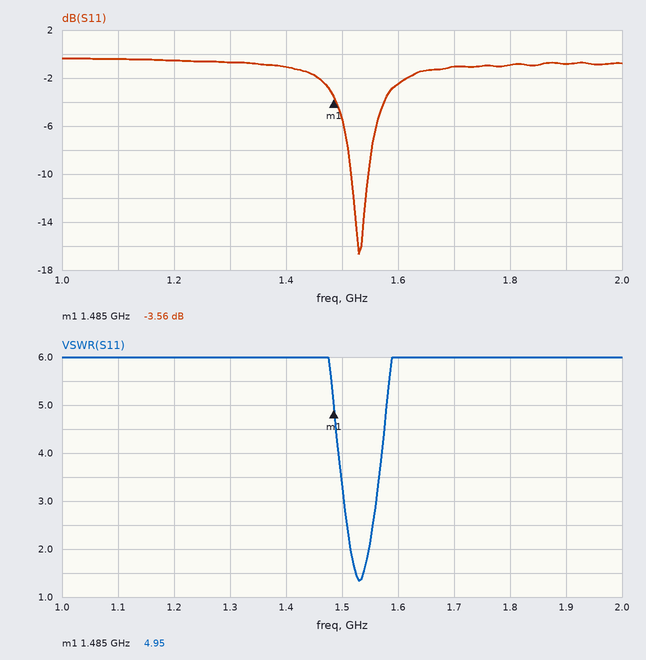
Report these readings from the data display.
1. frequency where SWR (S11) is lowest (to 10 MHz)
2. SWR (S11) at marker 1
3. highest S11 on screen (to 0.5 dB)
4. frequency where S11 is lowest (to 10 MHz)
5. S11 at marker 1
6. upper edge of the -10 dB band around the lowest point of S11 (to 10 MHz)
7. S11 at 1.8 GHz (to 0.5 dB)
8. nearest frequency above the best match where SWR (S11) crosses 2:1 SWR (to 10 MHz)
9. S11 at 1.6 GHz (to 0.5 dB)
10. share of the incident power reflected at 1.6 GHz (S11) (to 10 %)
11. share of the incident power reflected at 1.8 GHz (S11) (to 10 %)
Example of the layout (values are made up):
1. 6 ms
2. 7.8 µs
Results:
1. 1.53 GHz
2. 4.95
3. -0.5 dB
4. 1.53 GHz
5. -3.56 dB
6. 1.55 GHz
7. -1.0 dB
8. 1.55 GHz
9. -2.5 dB
10. 60 %
11. 80 %
